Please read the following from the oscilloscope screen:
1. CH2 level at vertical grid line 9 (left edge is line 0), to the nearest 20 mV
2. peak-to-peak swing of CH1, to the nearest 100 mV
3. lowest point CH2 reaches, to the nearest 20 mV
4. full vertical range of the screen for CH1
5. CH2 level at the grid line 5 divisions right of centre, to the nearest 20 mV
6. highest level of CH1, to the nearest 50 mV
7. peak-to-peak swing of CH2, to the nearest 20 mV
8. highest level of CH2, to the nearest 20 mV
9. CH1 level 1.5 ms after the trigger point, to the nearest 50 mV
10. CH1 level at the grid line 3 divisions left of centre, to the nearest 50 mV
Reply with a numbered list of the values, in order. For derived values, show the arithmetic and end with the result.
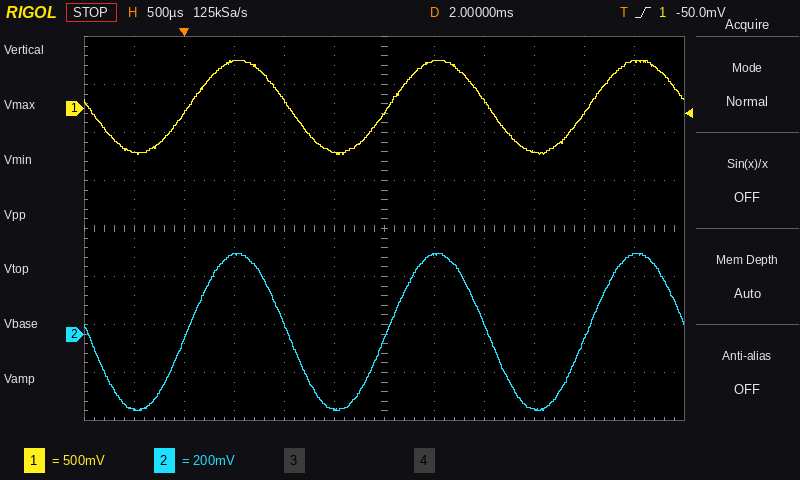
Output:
1. -320 mV
2. 1.00 V
3. -320 mV
4. 4 V
5. 340 mV
6. 500 mV
7. 340 mV − (-320 mV) = 660 mV
8. 340 mV
9. -450 mV
10. 500 mV
